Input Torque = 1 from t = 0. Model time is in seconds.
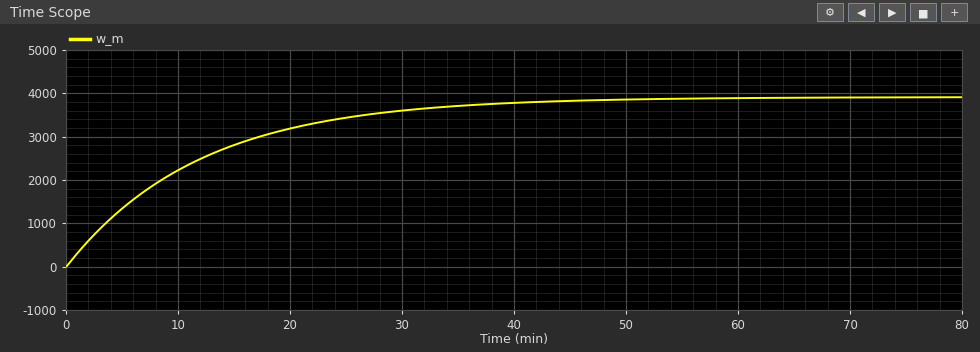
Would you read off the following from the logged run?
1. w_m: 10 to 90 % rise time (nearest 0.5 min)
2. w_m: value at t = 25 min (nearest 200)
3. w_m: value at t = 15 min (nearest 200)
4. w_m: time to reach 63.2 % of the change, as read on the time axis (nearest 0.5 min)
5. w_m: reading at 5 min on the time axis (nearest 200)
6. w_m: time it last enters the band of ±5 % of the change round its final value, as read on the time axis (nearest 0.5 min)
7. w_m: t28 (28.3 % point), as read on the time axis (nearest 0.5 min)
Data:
26.0 min
3400
2800
12.0 min
1400
35.5 min
4.0 min
